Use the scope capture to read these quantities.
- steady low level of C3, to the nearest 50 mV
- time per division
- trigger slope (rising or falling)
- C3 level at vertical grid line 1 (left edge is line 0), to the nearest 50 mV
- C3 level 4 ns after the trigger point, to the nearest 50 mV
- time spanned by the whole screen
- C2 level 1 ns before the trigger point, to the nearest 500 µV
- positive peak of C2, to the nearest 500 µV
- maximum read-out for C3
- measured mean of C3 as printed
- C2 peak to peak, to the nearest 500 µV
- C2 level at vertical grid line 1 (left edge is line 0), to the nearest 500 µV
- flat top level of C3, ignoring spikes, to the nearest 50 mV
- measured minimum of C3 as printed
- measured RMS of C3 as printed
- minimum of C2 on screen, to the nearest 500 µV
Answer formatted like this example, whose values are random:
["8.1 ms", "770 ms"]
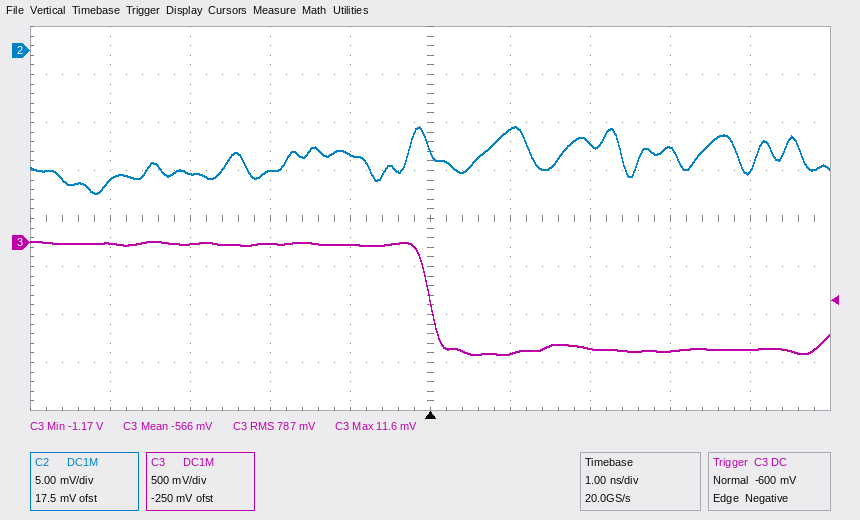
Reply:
["-1.10 V", "1 ns", "falling", "0 mV", "-1.10 V", "10 ns", "-11.0 mV", "-8.0 mV", "11.6 mV", "-566 mV", "7.0 mV", "-13.5 mV", "0 mV", "-1.17 V", "787 mV", "-15.0 mV"]
